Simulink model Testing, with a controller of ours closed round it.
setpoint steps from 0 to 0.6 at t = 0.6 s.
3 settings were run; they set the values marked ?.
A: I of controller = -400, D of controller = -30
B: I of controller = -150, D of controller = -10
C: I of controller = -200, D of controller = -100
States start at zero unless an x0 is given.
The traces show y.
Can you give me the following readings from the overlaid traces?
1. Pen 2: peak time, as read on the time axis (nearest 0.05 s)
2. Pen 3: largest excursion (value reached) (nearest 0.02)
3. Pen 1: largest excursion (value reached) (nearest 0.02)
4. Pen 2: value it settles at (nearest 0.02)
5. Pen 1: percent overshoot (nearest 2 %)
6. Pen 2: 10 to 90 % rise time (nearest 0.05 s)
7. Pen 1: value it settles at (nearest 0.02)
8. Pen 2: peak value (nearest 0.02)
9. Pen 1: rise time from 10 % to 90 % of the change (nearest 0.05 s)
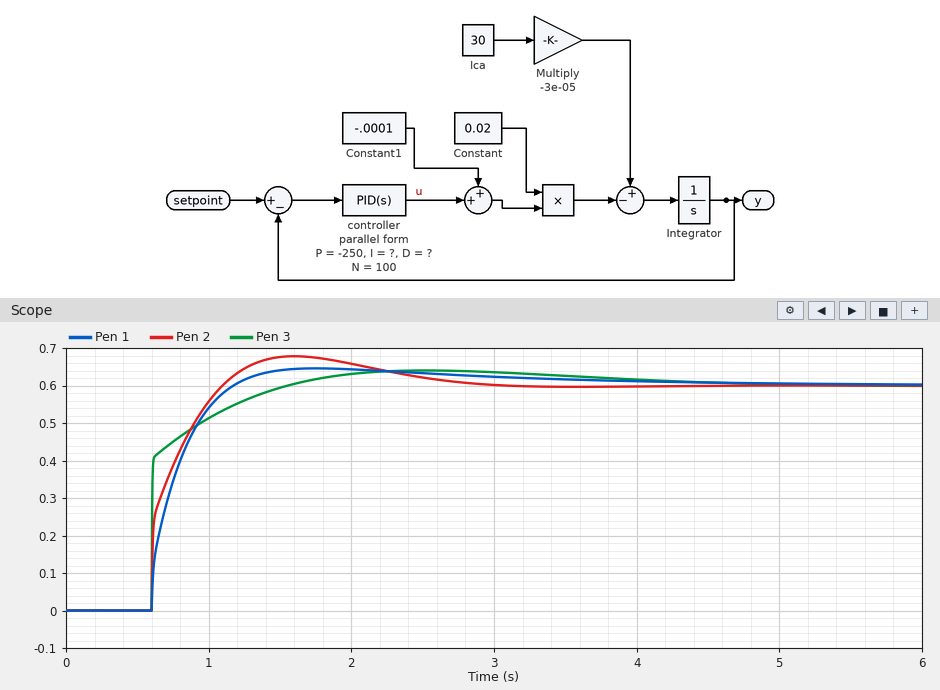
1.60 s
0.64
0.64
0.60
8 %
0.35 s
0.60
0.68
0.40 s
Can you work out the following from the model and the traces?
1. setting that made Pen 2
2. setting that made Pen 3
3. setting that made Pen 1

A
C
B
